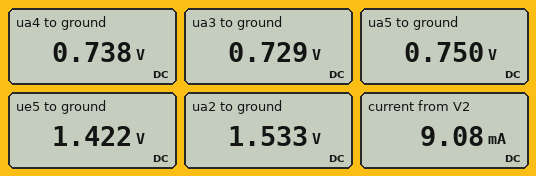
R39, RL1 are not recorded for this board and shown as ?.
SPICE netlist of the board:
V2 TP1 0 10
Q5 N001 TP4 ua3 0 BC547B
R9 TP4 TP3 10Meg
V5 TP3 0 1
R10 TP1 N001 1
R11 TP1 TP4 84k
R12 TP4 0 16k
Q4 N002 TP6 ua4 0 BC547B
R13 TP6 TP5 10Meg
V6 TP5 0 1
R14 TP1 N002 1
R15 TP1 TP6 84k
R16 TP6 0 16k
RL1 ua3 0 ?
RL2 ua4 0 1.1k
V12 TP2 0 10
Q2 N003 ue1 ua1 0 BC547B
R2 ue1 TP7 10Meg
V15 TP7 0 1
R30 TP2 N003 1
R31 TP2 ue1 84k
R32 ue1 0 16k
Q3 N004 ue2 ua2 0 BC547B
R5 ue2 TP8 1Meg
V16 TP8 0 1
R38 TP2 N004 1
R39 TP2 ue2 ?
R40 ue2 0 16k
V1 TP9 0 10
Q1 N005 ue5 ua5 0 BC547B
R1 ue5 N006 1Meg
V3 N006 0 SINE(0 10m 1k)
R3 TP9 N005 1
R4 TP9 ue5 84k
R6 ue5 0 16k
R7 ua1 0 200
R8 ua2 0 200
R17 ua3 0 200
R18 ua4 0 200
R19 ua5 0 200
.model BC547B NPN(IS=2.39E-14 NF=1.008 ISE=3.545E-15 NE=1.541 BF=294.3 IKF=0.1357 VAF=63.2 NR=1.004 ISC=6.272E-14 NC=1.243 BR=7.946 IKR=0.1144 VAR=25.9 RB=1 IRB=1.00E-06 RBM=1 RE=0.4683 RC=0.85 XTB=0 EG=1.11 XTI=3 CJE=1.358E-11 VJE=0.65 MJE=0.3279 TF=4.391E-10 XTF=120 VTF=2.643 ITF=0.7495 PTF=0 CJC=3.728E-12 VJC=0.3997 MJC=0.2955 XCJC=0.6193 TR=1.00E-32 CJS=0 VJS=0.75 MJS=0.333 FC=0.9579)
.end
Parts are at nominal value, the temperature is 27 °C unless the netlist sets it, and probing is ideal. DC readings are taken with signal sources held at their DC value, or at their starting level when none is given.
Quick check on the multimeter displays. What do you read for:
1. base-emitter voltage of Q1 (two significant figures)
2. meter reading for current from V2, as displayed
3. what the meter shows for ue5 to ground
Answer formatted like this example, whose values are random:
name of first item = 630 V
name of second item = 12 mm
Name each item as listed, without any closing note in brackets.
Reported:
base-emitter voltage of Q1 = 670 mV
meter reading for current from V2, as displayed = 9.08 mA
what the meter shows for ue5 to ground = 1.422 V
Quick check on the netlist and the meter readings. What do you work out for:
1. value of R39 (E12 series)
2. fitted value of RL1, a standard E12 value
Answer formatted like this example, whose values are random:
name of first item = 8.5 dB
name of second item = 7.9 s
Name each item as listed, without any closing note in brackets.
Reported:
value of R39 = 47 kΩ
fitted value of RL1, a standard E12 value = 820 Ω
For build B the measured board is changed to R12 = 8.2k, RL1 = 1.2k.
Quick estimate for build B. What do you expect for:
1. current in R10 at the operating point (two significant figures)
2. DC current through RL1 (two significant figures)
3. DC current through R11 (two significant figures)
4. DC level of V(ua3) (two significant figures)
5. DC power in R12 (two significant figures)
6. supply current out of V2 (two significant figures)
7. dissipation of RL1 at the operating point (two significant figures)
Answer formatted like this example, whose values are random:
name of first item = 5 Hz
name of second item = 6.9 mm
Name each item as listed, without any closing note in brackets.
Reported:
current in R10 at the operating point = 1.3 mA
DC current through RL1 = 180 µA
DC current through R11 = 110 µA
DC level of V(ua3) = 220 mV
DC power in R12 = 90 µW
supply current out of V2 = 5.8 mA
dissipation of RL1 at the operating point = 40 µW
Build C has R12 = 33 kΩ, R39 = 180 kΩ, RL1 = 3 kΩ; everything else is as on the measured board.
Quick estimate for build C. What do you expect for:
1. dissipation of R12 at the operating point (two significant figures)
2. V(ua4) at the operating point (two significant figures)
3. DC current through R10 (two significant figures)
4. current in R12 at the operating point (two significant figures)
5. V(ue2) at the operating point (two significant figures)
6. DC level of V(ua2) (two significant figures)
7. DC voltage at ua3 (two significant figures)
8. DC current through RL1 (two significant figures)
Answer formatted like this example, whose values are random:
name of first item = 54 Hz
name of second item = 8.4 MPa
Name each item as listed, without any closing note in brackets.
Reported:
dissipation of R12 at the operating point = 150 µW
V(ua4) at the operating point = 740 mV
DC current through R10 = 8.0 mA
current in R12 at the operating point = 67 µA
V(ue2) at the operating point = 780 mV
DC level of V(ua2) = 160 mV
DC voltage at ua3 = 1.5 V
DC current through RL1 = 500 µA
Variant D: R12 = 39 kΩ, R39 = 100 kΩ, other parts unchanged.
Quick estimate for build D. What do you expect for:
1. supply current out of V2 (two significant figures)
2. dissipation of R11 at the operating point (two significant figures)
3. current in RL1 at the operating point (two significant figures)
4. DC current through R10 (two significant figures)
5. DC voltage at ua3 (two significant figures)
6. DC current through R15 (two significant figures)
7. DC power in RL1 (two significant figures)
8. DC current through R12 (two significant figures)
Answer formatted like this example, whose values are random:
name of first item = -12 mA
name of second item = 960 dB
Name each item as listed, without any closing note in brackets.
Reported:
supply current out of V2 = 14 mA
dissipation of R11 at the operating point = 710 µW
current in RL1 at the operating point = 1.9 mA
DC current through R10 = 9.9 mA
DC voltage at ua3 = 1.6 V
DC current through R15 = 100 µA
DC power in RL1 = 3.1 mW
DC current through R12 = 59 µA
